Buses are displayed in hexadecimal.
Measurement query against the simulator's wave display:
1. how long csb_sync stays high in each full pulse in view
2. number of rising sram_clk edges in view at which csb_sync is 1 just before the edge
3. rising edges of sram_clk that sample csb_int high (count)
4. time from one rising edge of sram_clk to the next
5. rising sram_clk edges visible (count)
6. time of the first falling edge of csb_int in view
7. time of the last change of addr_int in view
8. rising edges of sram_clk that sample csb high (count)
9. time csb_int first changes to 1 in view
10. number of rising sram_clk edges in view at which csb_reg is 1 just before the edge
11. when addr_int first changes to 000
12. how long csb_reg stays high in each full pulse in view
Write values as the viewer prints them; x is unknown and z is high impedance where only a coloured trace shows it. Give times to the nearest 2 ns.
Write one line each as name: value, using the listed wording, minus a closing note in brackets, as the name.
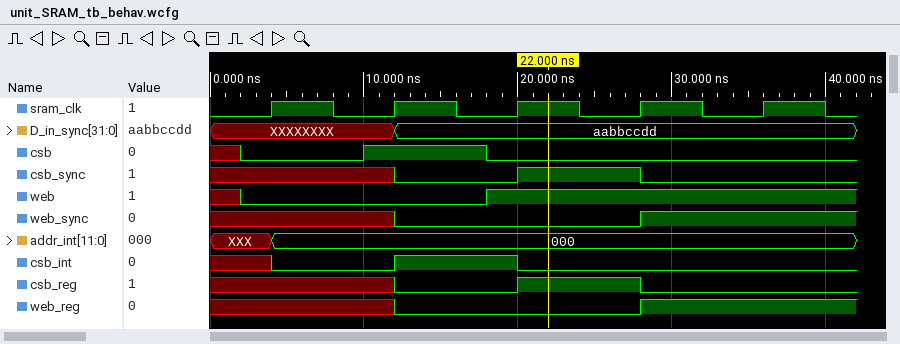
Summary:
how long csb_sync stays high in each full pulse in view: 8 ns
number of rising sram_clk edges in view at which csb_sync is 1 just before the edge: 1
rising edges of sram_clk that sample csb_int high: 1
time from one rising edge of sram_clk to the next: 8 ns
rising sram_clk edges visible: 5
time of the first falling edge of csb_int in view: 20 ns
time of the last change of addr_int in view: 4 ns
rising edges of sram_clk that sample csb high: 1
time csb_int first changes to 1 in view: 12 ns
number of rising sram_clk edges in view at which csb_reg is 1 just before the edge: 1
when addr_int first changes to 000: 4 ns
how long csb_reg stays high in each full pulse in view: 8 ns
